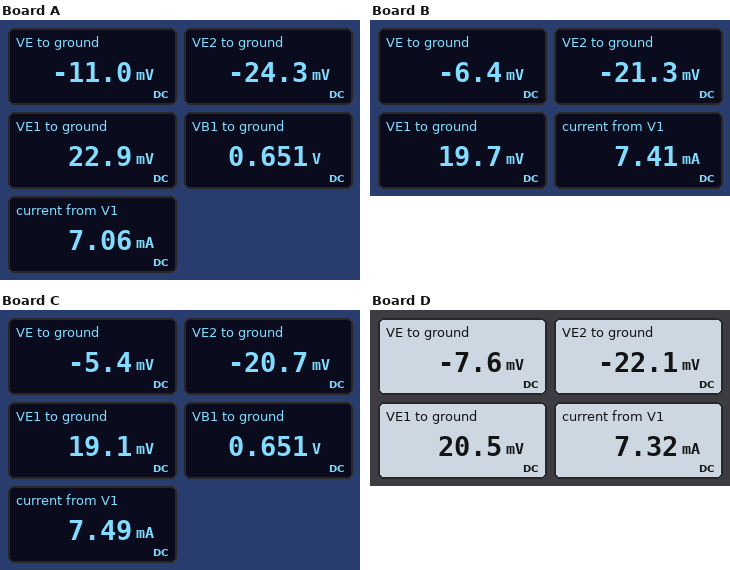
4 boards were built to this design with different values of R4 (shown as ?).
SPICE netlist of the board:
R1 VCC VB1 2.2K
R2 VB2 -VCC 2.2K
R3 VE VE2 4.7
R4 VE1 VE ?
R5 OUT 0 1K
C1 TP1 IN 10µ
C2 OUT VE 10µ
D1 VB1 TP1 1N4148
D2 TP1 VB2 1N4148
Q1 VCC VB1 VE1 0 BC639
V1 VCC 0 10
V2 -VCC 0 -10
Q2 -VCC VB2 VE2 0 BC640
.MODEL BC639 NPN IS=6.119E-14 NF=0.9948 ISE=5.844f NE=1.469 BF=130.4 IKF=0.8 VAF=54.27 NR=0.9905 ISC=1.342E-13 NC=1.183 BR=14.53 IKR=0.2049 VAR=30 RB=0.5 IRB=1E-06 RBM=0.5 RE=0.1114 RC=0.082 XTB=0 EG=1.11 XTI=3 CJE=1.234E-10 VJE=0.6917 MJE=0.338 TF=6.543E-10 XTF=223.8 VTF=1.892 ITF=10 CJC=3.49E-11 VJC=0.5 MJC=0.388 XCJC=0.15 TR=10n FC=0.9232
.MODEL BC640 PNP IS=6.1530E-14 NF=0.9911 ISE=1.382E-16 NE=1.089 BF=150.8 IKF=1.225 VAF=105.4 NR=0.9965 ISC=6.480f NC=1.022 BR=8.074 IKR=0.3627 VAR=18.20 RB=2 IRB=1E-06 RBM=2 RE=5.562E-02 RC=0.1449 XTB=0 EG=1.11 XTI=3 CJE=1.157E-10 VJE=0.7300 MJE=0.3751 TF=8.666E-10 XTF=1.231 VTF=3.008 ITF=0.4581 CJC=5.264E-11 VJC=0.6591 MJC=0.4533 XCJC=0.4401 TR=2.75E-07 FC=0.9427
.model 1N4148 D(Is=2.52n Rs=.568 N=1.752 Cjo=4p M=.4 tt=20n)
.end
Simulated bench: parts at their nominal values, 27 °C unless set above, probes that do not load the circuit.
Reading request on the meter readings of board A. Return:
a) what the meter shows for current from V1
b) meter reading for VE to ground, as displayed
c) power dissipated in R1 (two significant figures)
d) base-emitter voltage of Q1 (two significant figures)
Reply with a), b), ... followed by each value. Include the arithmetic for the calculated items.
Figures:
a) 7.06 mA
b) -11.0 mV
c) (10 V - 651 mV)^2 / 2.2 kΩ = 40 mW
d) 651 mV - 22.9 mV = 630 mV
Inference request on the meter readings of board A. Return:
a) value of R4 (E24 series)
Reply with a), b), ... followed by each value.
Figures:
a) 12 Ω
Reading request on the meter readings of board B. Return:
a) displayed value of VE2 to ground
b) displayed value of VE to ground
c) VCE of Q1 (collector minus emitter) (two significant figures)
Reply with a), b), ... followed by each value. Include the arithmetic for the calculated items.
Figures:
a) -21.3 mV
b) -6.4 mV
c) 10 V - 19.7 mV = 10 V
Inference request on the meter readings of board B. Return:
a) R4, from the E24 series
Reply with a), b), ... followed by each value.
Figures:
a) 8.2 Ω
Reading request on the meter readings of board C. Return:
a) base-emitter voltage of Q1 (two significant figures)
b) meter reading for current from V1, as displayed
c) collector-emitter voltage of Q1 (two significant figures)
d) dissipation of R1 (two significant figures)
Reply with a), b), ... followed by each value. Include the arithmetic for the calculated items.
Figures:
a) 651 mV - 19.1 mV = 630 mV
b) 7.49 mA
c) 10 V - 19.1 mV = 10 V
d) (10 V - 651 mV)^2 / 2.2 kΩ = 40 mW
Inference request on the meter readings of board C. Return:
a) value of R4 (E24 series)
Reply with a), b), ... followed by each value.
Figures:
a) 7.5 Ω
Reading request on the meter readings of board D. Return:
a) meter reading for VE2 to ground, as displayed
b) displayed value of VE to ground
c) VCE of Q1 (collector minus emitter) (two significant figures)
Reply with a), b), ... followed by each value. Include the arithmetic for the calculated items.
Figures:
a) -22.1 mV
b) -7.6 mV
c) 10 V - 20.5 mV = 10 V
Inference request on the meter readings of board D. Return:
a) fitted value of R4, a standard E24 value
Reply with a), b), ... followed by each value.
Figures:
a) 9.1 Ω
